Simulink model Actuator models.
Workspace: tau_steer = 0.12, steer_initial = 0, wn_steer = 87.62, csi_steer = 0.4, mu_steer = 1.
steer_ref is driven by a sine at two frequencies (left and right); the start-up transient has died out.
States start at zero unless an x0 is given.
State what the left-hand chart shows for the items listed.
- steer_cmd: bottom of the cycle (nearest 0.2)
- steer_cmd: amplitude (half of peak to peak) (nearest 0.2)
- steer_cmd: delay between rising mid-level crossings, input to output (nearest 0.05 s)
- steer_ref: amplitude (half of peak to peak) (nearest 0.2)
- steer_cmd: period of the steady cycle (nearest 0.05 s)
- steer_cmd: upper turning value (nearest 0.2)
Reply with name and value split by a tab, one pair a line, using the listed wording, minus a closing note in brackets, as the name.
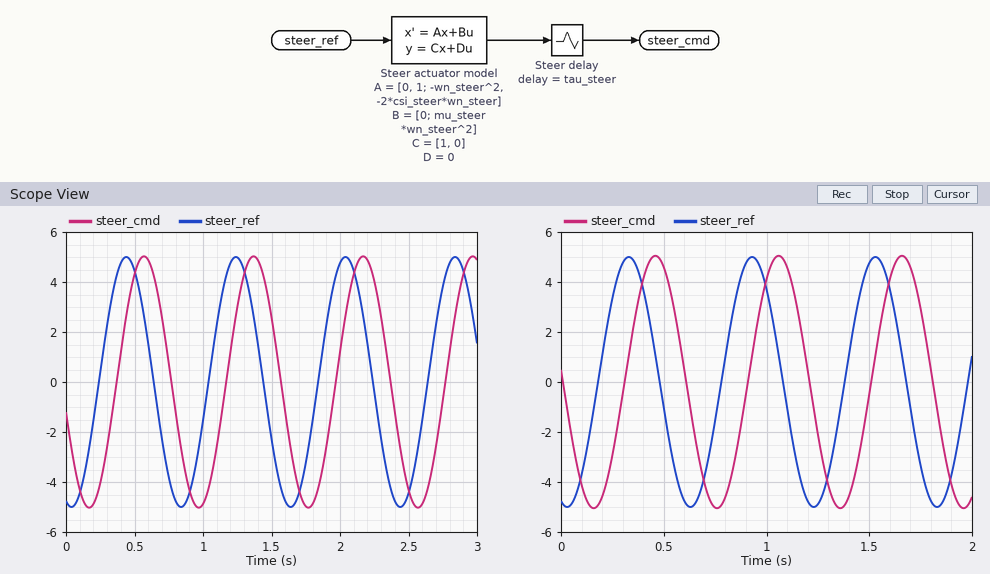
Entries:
steer_cmd: bottom of the cycle	-5.0
steer_cmd: amplitude (half of peak to peak)	5.0
steer_cmd: delay between rising mid-level crossings, input to output	0.15 s
steer_ref: amplitude (half of peak to peak)	5.0
steer_cmd: period of the steady cycle	0.80 s
steer_cmd: upper turning value	5.0
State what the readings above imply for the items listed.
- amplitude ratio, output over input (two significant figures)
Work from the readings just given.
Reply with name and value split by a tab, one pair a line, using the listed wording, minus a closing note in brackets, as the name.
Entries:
amplitude ratio, output over input	1.0
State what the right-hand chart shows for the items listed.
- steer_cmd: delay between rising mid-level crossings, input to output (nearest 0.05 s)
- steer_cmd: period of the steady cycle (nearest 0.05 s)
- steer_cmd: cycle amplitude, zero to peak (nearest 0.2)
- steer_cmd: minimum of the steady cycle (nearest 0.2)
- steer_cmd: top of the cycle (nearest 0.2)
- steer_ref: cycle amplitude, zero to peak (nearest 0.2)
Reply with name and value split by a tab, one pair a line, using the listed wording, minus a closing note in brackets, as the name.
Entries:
steer_cmd: delay between rising mid-level crossings, input to output	0.15 s
steer_cmd: period of the steady cycle	0.60 s
steer_cmd: cycle amplitude, zero to peak	5.0
steer_cmd: minimum of the steady cycle	-5.0
steer_cmd: top of the cycle	5.0
steer_ref: cycle amplitude, zero to peak	5.0
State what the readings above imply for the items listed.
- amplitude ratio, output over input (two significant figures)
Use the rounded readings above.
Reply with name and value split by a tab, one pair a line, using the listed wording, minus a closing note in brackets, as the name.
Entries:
amplitude ratio, output over input	1.0
